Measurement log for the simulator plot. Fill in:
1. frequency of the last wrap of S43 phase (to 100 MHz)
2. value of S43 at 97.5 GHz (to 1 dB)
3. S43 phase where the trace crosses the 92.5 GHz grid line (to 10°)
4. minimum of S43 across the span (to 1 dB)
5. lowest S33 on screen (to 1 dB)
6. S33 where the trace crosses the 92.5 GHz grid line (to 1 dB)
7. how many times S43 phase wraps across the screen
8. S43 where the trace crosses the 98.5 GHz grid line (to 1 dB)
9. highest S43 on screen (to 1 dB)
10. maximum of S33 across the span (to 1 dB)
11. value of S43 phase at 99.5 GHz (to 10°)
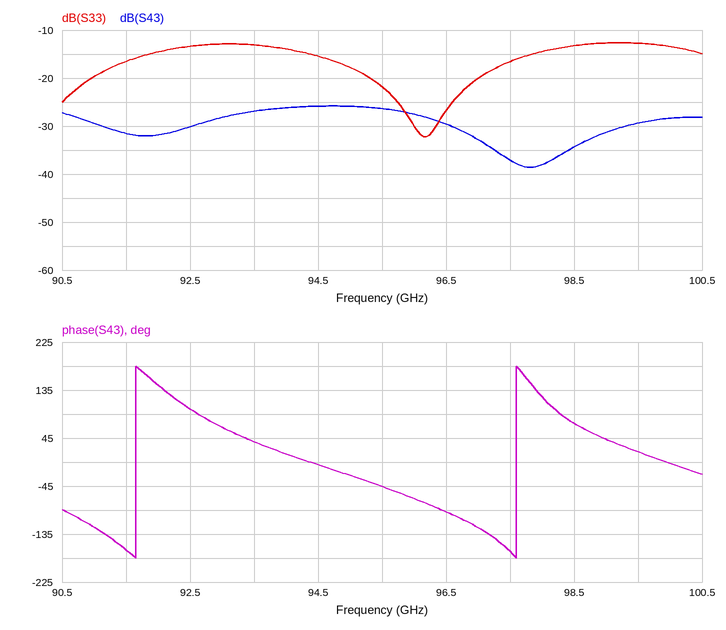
97.6 GHz
-37 dB
100°
-39 dB
-32 dB
-13 dB
2
-34 dB
-26 dB
-13 dB
20°
